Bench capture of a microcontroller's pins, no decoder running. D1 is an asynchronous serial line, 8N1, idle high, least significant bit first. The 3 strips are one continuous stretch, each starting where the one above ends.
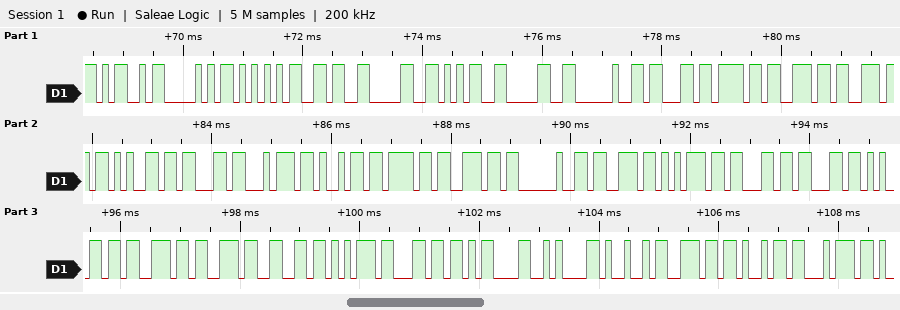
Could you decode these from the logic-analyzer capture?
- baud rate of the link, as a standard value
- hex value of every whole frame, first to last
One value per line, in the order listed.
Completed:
9600 baud
4D 50 55 36 30 35 30 20 63 6F 6E 6E 65 63 74 69 6F 6E 20 73 75 63 63 65 73 73 66 75 6C 0D 0A 49 6E 69 74
